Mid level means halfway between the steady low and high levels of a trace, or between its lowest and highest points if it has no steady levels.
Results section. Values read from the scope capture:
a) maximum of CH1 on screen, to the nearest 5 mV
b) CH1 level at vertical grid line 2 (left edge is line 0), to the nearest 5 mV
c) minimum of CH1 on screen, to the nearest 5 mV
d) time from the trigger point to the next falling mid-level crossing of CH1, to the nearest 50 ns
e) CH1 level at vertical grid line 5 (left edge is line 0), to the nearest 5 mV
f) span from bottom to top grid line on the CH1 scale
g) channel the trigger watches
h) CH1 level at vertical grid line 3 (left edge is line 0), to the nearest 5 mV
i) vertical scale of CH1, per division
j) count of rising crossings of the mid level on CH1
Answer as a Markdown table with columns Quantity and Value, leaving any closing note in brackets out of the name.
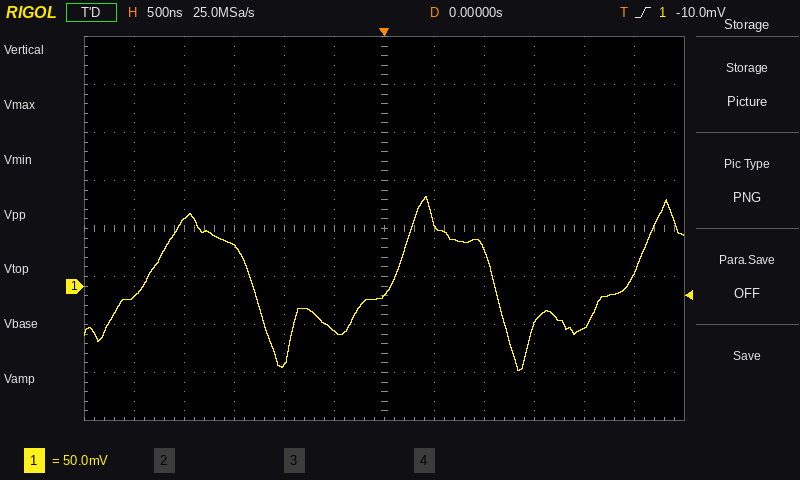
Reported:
| Quantity | Value |
|---|---|
| maximum of CH1 on screen, to the nearest 5 mV | 95 mV |
| CH1 level at vertical grid line 2 (left edge is line 0), to the nearest 5 mV | 70 mV |
| minimum of CH1 on screen, to the nearest 5 mV | -90 mV |
| time from the trigger point to the next falling mid-level crossing of CH1, to the nearest 50 ns | 1.10 µs |
| CH1 level at vertical grid line 5 (left edge is line 0), to the nearest 5 mV | -45 mV |
| span from bottom to top grid line on the CH1 scale | 400 mV |
| channel the trigger watches | CH1 |
| CH1 level at vertical grid line 3 (left edge is line 0), to the nearest 5 mV | 40 mV |
| vertical scale of CH1, per division | 50 mV |
| count of rising crossings of the mid level on CH1 | 3 |
